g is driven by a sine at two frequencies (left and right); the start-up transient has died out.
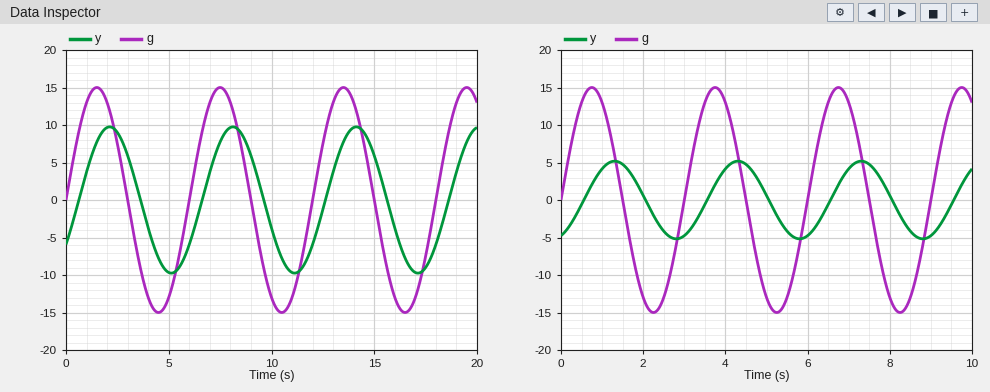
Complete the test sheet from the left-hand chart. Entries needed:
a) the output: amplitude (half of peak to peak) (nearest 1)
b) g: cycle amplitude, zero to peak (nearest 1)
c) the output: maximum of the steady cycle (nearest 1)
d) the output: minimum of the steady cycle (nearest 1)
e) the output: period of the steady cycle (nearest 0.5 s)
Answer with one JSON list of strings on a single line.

["10", "15", "10", "-10", "6.0 s"]
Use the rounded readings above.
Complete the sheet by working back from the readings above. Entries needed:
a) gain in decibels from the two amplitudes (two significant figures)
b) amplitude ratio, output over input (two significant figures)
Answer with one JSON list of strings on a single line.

["-3.5 dB", "0.67"]
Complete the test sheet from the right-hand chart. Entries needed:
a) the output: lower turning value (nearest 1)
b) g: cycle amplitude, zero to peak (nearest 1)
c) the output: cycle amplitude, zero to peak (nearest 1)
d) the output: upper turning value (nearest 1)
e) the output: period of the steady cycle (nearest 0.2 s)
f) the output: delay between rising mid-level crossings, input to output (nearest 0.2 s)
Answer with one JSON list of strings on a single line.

["-5", "15", "5", "5", "3.0 s", "0.6 s"]
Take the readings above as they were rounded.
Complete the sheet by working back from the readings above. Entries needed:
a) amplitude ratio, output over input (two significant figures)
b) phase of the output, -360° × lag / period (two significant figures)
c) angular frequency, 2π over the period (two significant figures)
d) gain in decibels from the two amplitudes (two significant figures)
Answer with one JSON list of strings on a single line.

["0.33", "-72°", "2.1 rad/s", "-9.5 dB"]
